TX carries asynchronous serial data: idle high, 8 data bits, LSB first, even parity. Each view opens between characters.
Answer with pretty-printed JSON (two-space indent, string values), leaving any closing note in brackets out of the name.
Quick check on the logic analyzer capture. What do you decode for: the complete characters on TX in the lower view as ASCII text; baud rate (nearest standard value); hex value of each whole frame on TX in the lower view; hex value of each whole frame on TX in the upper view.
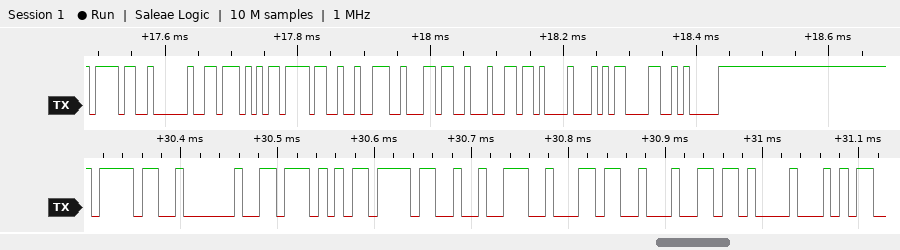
{
  "the complete characters on TX in the lower view as ASCII text": "\"o World!\"",
  "baud rate": "115200 baud",
  "hex value of each whole frame on TX in the lower view": "6F, 20, 57, 6F, 72, 6C, 64, 21",
  "hex value of each whole frame on TX in the upper view": "6F, 20, 57, 6F, 72, 6C, 64, 21, 0D, 0A"
}
